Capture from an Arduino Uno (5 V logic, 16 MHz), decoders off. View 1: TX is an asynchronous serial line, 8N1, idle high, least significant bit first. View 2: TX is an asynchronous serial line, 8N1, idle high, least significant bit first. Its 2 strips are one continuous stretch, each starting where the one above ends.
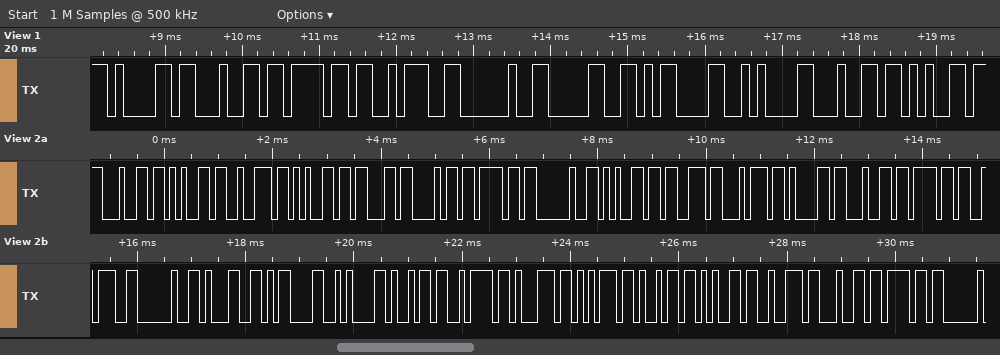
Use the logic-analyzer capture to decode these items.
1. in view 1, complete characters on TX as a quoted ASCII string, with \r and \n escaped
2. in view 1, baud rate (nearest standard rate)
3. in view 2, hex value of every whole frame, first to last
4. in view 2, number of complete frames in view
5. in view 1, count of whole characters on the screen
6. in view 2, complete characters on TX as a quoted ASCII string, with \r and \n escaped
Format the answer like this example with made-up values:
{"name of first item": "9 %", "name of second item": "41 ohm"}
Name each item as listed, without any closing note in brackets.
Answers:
{"in view 1, complete characters on TX as a quoted ASCII string, with \\r and \\n escaped": "\"ado: 0\\r\\nde\"", "in view 1, baud rate": "9600 baud", "in view 2, hex value of every whole frame, first to last": "0x64 0x65 0x72 0x65 0x63 0x68 0x6F 0x20 0x65 0x73 0x74 0x61 0x64 0x6F 0x3A 0x20 0x31 0x0D 0x0A 0x69 0x7A 0x71 0x75 0x69 0x65 0x72 0x64 0x6F", "in view 2, number of complete frames in view": "28", "in view 1, count of whole characters on the screen": "10", "in view 2, complete characters on TX as a quoted ASCII string, with \\r and \\n escaped": "\"derecho estado: 1\\r\\nizquierdo\""}
